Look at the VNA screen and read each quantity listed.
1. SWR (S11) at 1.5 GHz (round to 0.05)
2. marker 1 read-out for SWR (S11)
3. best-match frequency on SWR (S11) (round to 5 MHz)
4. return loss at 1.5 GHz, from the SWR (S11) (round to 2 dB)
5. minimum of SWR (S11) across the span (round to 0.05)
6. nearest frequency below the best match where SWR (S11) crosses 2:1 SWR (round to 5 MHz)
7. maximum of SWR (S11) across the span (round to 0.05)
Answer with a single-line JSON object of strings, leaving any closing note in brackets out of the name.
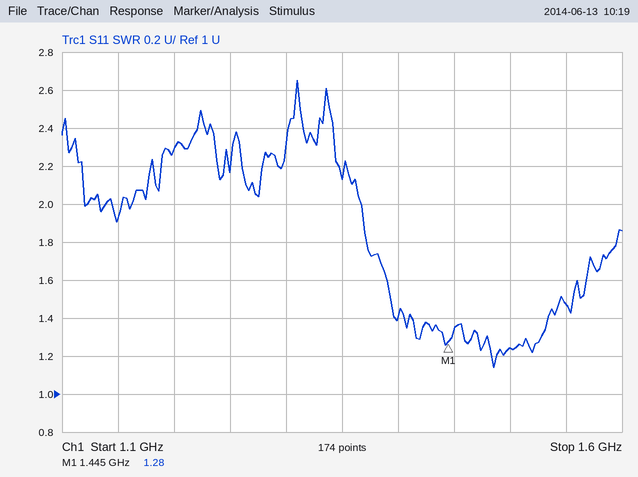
{"SWR (S11) at 1.5 GHz": "1.25", "marker 1 read-out for SWR": "1.28", "best-match frequency on SWR (S11)": "1.485 GHz", "return loss at 1.5 GHz, from the SWR (S11)": "20 dB", "minimum of SWR (S11) across the span": "1.15", "nearest frequency below the best match where SWR (S11) crosses 2:1 SWR": "1.365 GHz", "maximum of SWR (S11) across the span": "2.65"}
